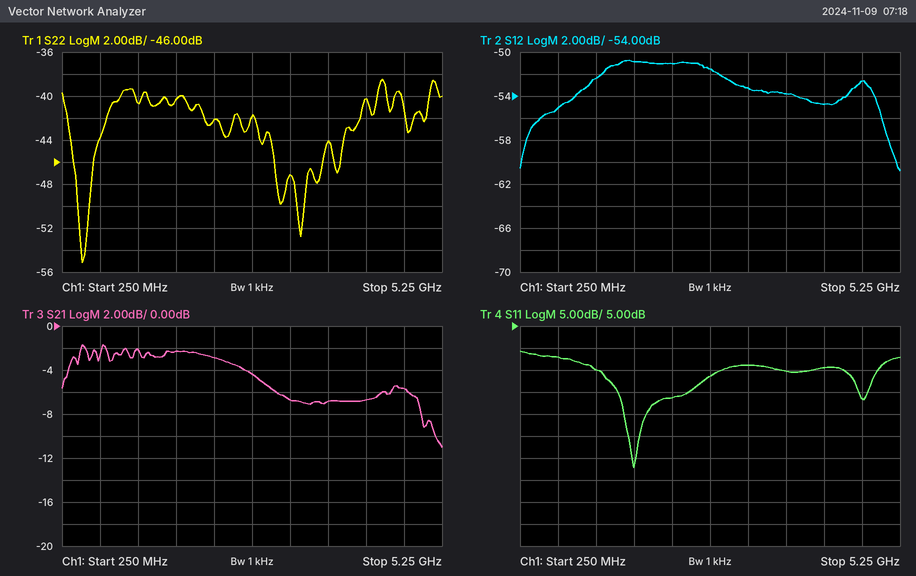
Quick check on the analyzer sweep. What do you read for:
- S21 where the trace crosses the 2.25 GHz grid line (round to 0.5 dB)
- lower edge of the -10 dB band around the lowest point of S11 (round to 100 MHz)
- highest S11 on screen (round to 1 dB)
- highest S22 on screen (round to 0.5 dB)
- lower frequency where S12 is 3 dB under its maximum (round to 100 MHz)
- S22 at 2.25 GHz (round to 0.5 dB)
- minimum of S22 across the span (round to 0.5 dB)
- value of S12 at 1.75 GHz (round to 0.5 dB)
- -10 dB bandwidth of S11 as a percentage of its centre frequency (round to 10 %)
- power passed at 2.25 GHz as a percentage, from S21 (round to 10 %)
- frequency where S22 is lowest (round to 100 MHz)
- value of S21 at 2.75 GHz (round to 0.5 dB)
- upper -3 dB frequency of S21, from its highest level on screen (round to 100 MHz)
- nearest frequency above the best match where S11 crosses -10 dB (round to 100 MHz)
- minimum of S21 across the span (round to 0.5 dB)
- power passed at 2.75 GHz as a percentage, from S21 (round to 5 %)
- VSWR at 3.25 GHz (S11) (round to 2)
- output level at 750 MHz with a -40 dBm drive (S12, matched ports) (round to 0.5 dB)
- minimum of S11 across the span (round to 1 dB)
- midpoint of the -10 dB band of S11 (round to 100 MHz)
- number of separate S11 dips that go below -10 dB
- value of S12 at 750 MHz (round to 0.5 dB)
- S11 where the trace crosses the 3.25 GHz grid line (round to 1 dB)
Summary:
-3.0 dB
1.5 GHz
-1 dB
-38.5 dB
1.0 GHz
-42.0 dB
-55.0 dB
-51.0 dB
50 %
50 %
500 MHz
-4.5 dB
2.8 GHz
2.5 GHz
-11.0 dB
35 %
4
-95.0 dBm
-27 dB
2.0 GHz
2
-55.0 dB
-4 dB
